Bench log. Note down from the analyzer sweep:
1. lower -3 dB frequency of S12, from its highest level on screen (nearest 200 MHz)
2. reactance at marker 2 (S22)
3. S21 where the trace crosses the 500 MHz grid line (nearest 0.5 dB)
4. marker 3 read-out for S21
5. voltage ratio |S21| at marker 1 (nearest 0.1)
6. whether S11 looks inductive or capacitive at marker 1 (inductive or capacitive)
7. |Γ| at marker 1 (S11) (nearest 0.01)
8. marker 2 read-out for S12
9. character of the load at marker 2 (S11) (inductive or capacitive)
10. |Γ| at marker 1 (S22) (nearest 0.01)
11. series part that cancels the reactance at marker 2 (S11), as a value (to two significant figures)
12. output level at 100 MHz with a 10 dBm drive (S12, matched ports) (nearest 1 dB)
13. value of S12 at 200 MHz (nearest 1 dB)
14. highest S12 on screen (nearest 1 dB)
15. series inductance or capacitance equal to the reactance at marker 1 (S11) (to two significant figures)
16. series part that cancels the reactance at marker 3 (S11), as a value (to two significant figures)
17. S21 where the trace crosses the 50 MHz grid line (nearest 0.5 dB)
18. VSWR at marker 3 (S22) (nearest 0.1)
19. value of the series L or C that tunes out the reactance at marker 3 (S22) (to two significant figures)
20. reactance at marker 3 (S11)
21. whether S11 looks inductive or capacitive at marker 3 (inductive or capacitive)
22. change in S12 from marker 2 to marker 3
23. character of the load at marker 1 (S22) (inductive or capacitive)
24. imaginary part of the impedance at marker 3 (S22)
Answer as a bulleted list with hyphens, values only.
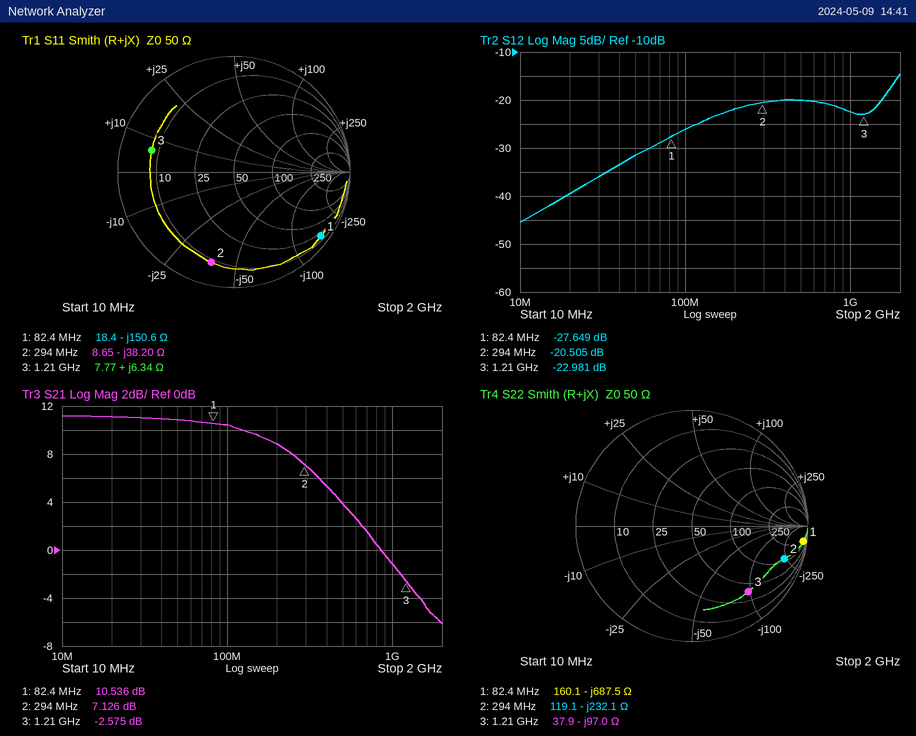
- 1.8 GHz
- -232.1 Ω
- 4.0 dB
- -2.575 dB
- 3.4
- capacitive
- 0.93
- -20.505 dB
- capacitive
- 0.97
- 21 nH
- -16 dBm
- -22 dB
- -15 dB
- 13 pF
- 21 pF
- 11.0 dB
- 6.9
- 13 nH
- +6.34 Ω
- inductive
- -2.476 dB
- capacitive
- -97.0 Ω
